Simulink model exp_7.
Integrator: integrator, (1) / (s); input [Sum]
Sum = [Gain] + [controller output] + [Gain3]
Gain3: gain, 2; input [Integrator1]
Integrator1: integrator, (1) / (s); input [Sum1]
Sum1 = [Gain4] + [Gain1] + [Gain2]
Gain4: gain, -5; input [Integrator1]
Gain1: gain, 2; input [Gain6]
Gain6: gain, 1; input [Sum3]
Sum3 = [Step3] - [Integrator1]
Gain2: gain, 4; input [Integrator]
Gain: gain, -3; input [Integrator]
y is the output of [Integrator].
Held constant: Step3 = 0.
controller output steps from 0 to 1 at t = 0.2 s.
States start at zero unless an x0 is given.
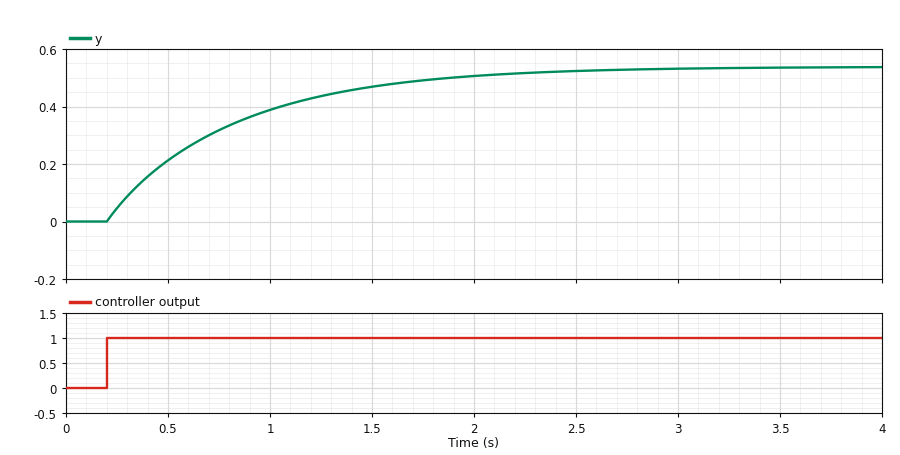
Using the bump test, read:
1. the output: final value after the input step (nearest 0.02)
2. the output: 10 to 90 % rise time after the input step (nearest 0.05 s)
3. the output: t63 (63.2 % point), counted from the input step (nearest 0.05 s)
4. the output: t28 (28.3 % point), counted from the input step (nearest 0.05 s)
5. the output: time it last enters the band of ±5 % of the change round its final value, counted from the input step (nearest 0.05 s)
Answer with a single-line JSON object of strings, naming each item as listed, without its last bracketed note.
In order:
{"the output: final value after the input step": "0.54", "the output: 10 to 90 % rise time after the input step": "1.40 s", "the output: t63 (63.2 % point), counted from the input step": "0.60 s", "the output: t28 (28.3 % point), counted from the input step": "0.20 s", "the output: time it last enters the band of ±5 % of the change round its final value, counted from the input step": "1.90 s"}
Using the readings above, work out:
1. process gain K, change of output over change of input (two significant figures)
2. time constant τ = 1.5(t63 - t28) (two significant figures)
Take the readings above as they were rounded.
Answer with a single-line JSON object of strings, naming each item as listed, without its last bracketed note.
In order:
{"process gain K, change of output over change of input": "0.54", "time constant τ = 1.5(t63 - t28)": "0.60 s"}
